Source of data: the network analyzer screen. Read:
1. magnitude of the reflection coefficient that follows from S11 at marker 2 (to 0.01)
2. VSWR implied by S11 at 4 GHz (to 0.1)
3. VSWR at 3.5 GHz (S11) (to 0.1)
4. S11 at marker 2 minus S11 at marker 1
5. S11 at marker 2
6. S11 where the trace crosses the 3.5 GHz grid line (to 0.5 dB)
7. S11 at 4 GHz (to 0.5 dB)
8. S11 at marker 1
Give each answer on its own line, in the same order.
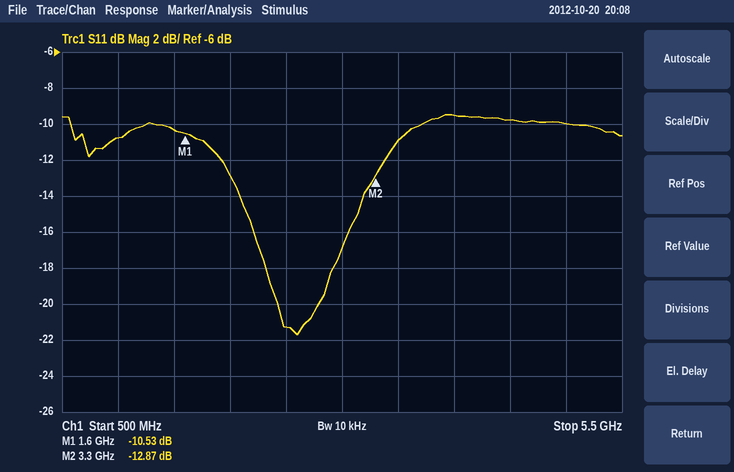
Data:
0.23
2.0
1.8
-2.34 dB
-12.87 dB
-11.0 dB
-9.5 dB
-10.53 dB
